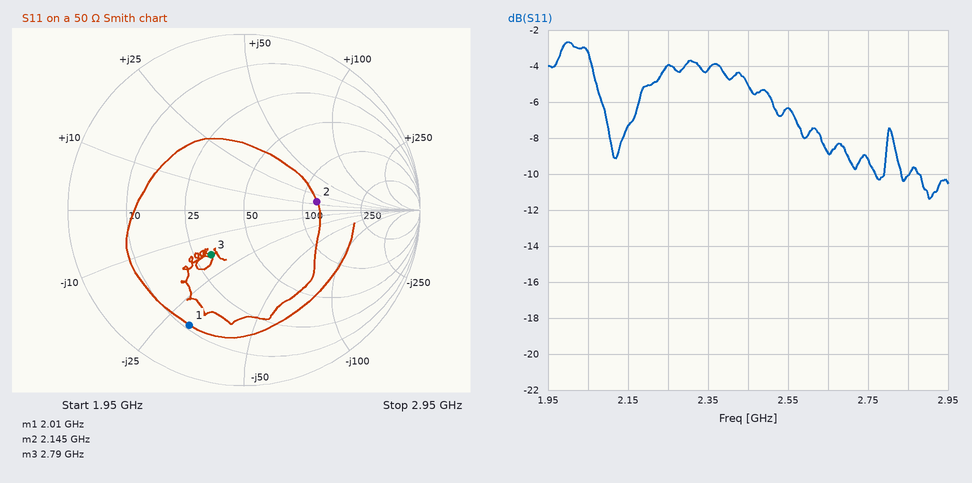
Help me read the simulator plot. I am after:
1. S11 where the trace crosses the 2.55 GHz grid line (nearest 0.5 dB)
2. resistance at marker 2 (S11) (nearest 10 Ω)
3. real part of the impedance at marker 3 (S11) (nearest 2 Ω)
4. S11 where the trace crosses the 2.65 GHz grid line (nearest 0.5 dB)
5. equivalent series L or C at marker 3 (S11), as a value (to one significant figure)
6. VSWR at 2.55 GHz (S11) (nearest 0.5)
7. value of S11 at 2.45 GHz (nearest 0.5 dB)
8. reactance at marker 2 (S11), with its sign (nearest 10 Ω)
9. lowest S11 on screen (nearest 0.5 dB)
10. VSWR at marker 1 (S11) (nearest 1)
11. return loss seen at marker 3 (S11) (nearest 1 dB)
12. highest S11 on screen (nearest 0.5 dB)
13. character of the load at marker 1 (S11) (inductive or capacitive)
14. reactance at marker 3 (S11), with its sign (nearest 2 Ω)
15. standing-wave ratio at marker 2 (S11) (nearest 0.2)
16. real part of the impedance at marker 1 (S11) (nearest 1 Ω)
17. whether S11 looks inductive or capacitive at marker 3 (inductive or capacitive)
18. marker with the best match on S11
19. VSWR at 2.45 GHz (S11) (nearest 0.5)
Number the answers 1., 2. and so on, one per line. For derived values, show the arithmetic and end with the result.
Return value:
1. -6.5 dB
2. 120 Ω
3. 30 Ω
4. -9.0 dB
5. C = 1/(2π × 2.79 GHz × 18 Ω) ≈ 3 pF
6. |Γ| = 10^(-6.5/20) = 0.4732; VSWR = (1 + 0.4732)/(1 − 0.4732) ≈ 2.80, so 3.0 to the nearest 0.5
7. -5.0 dB
8. +10 Ω
9. -11.5 dB
10. 6
11. 10 dB
12. -2.5 dB
13. capacitive
14. -18 Ω
15. 2.4
16. 11 Ω
17. capacitive
18. marker 3
19. |Γ| = 10^(-5/20) = 0.5623; VSWR = (1 + 0.5623)/(1 − 0.5623) ≈ 3.57, so 3.5 to the nearest 0.5
